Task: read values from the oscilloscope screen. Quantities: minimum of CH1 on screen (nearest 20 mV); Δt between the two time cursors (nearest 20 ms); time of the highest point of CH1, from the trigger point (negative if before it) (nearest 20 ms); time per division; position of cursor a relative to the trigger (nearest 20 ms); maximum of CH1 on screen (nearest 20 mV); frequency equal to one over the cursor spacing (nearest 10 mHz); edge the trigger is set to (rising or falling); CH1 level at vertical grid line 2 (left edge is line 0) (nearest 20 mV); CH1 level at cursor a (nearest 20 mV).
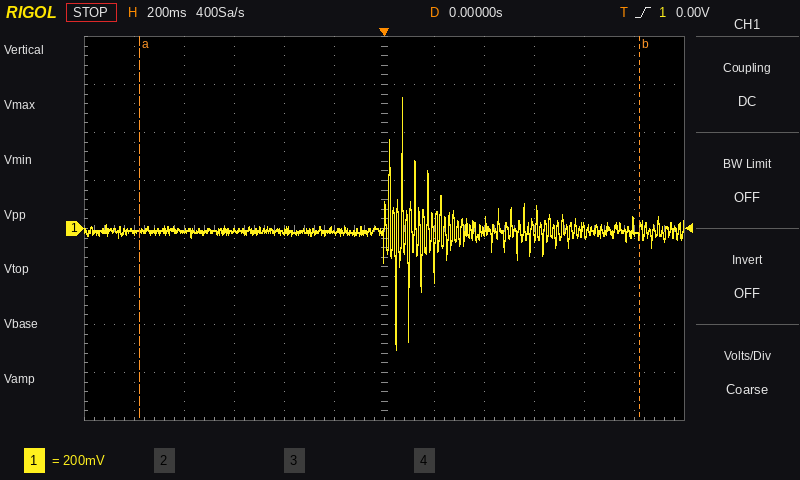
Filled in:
-500 mV
2.00 s
+80 ms
200 ms
-980 ms
540 mV
500 mHz
rising
0 mV
0 mV
